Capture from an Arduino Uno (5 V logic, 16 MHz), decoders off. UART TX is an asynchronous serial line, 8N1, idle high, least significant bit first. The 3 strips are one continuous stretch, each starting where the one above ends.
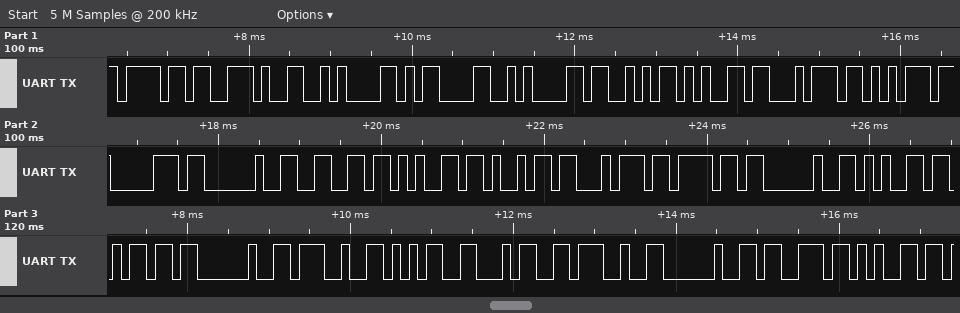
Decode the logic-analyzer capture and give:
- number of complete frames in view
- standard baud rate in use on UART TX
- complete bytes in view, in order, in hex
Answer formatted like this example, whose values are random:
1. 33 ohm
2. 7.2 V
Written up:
1. 27
2. 9600 baud
3. 6F 2E 0A 0D 0A 53 65 74 75 70 20 66 65 69 74 6F 20 65 6D 20 27 35 34 27 20 73 65
